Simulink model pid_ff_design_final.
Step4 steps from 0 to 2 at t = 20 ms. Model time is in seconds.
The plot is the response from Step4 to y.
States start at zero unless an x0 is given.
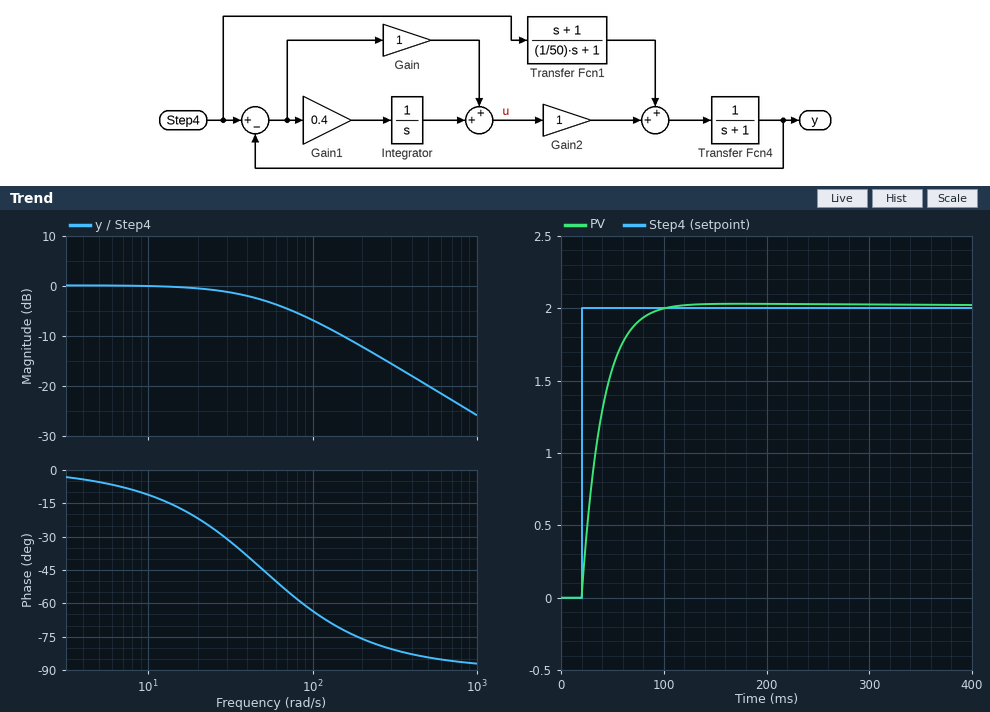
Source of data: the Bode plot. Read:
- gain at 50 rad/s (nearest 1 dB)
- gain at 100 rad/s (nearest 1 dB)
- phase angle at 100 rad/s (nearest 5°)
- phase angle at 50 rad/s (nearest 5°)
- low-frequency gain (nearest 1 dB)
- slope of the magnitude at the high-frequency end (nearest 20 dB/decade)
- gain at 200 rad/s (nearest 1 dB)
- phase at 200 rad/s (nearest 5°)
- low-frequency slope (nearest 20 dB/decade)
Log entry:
-3 dB
-7 dB
-65°
-45°
0 dB
-20 dB/decade
-12 dB
-75°
0 dB/decade
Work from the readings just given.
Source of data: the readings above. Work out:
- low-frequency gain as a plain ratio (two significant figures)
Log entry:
1.0
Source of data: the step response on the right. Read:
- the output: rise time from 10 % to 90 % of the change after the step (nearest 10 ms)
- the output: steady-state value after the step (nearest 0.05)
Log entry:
40 ms
2.00
